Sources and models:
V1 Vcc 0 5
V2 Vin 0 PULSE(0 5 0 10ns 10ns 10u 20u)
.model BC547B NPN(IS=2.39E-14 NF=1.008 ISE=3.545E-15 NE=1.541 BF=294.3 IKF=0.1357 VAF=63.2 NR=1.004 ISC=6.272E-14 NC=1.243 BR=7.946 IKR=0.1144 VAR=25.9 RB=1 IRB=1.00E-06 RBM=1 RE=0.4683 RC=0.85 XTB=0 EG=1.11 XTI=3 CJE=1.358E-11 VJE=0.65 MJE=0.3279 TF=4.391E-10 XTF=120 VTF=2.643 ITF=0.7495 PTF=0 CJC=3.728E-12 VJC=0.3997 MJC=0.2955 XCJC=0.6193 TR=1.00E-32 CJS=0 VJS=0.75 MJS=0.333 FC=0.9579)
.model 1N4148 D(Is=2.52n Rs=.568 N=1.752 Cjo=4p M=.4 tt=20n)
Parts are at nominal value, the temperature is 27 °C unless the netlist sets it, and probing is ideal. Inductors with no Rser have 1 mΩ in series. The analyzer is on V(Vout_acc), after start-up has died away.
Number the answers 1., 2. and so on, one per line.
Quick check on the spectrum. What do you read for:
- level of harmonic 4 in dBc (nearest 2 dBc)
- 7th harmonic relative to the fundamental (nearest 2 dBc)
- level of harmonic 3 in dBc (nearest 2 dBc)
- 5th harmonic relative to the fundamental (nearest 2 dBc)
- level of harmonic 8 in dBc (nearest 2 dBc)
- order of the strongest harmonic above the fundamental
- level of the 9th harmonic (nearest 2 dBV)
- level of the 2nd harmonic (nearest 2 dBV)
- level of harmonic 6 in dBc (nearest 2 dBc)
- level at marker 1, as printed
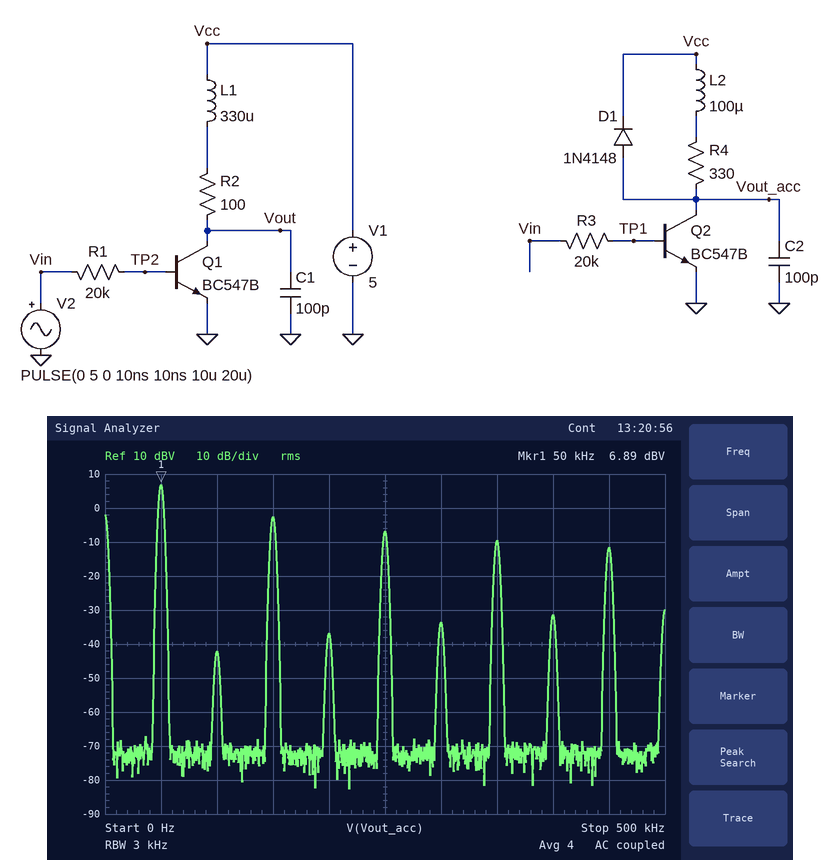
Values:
1. -44 dBc
2. -16 dBc
3. -10 dBc
4. -14 dBc
5. -38 dBc
6. 3
7. -12 dBV
8. -42 dBV
9. -40 dBc
10. 6.89 dBV
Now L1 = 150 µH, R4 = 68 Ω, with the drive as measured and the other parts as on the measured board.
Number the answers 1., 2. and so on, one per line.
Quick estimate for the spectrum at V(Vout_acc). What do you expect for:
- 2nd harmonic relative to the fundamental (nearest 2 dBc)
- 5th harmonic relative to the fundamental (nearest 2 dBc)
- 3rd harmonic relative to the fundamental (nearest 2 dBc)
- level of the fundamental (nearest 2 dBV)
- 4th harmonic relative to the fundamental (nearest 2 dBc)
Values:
1. -26 dBc
2. -10 dBc
3. -6 dBc
4. 4 dBV
5. -24 dBc
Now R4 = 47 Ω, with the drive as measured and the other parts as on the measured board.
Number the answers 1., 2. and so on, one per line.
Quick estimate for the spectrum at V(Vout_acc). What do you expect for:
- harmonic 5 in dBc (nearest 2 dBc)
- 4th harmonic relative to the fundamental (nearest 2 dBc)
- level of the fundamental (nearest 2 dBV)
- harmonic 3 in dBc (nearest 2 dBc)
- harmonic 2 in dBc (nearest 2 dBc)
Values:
1. -8 dBc
2. -16 dBc
3. 2 dBV
4. -6 dBc
5. -18 dBc
